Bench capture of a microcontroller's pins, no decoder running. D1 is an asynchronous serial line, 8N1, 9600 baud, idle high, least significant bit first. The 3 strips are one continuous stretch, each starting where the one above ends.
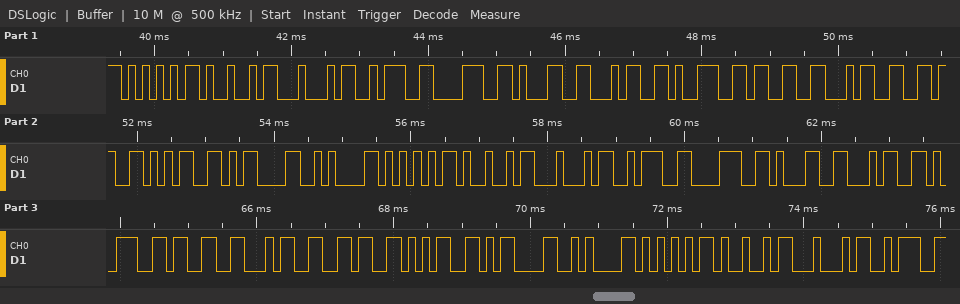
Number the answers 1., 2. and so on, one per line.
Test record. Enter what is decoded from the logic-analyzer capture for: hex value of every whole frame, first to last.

1. 0x55 0x49 0x44 0x3A 0x38 0x31 0x34 0x39 0x33 0x34 0x36 0x35 0x0D 0x0A 0x55 0x49 0x44 0x3A 0x38 0x31 0x34 0x39 0x33 0x34 0x36 0x35 0x0D 0x0A 0x55 0x49 0x44 0x3A
